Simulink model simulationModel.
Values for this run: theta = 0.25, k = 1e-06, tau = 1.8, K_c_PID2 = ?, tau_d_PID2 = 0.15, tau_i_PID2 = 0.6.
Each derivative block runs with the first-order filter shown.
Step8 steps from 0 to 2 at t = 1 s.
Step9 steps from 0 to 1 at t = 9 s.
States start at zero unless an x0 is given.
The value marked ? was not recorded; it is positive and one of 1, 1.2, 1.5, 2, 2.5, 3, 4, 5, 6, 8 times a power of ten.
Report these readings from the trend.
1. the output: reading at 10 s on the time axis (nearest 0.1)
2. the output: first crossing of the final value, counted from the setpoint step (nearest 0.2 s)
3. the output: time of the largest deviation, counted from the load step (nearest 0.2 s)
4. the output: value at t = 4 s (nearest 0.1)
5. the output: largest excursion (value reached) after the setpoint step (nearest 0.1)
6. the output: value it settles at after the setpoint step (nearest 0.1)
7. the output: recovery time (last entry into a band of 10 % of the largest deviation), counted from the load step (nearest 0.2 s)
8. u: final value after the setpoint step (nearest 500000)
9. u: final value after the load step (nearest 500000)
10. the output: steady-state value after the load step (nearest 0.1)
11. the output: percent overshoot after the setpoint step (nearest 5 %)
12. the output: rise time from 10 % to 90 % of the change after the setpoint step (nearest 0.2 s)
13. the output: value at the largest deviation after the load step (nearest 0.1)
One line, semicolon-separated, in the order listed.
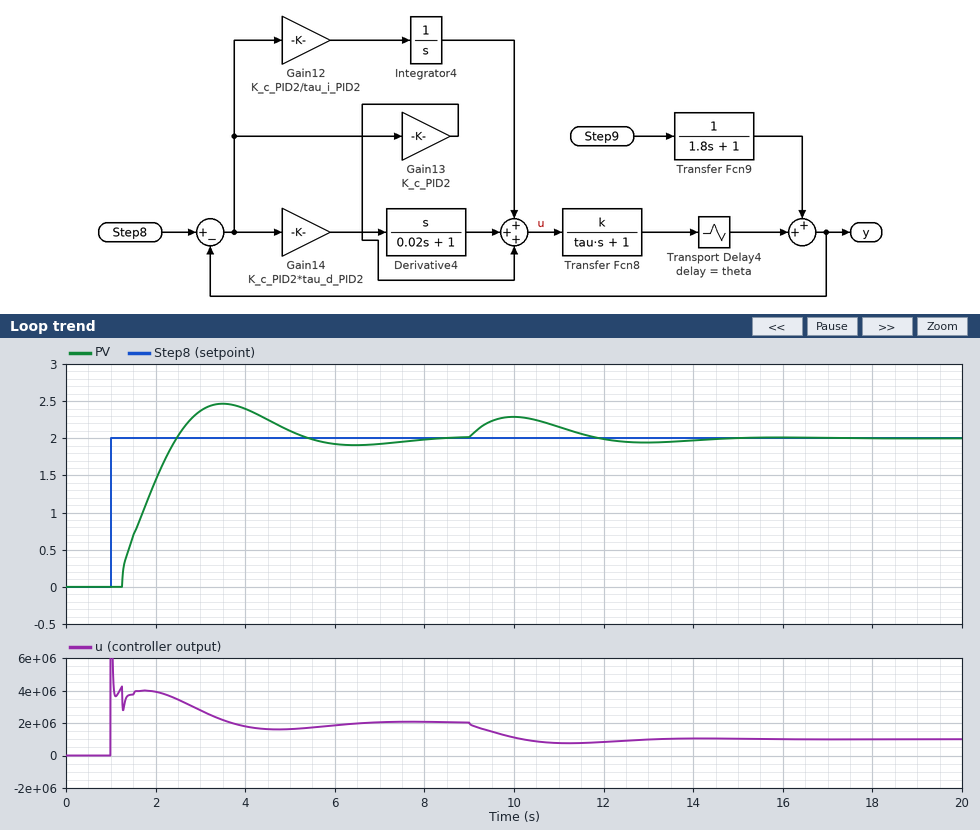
2.3; 1.4 s; 1.0 s; 2.4; 2.5; 2.0; 5.0 s; 2000000; 1000000; 2.0; 25 %; 1.0 s; 2.3
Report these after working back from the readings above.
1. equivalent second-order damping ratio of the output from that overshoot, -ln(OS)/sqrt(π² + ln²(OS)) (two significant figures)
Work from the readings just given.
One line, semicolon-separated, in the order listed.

0.40
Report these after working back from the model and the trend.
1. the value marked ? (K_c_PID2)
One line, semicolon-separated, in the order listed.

1.5e+06
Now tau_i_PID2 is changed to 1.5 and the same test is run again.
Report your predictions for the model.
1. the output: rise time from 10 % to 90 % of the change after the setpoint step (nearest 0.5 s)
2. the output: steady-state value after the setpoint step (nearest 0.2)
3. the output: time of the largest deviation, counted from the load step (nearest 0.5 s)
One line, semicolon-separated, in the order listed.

2.0 s; 2.0; 1.5 s
